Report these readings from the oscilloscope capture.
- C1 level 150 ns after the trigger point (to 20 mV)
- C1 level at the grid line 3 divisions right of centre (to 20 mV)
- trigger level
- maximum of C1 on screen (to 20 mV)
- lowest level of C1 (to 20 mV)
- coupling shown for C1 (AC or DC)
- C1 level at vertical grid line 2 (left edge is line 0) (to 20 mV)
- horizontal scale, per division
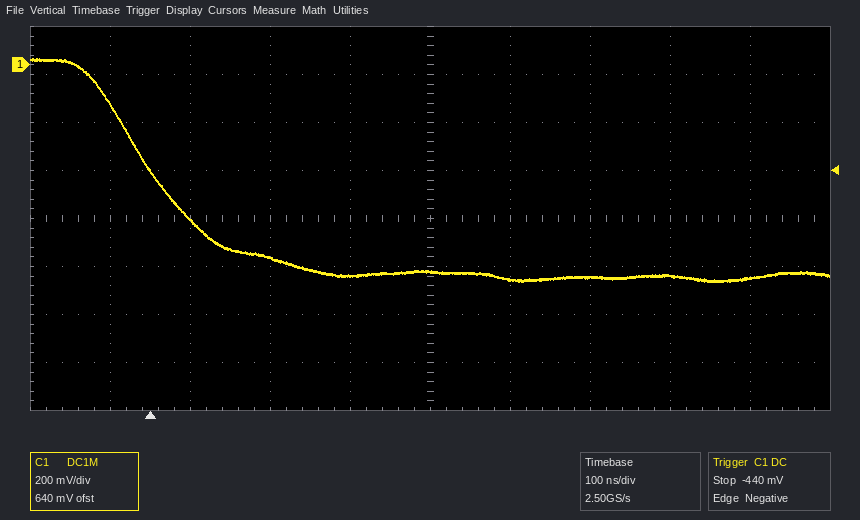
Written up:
-800 mV
-880 mV
-440 mV
20 mV
-900 mV
DC
-640 mV
100 ns
